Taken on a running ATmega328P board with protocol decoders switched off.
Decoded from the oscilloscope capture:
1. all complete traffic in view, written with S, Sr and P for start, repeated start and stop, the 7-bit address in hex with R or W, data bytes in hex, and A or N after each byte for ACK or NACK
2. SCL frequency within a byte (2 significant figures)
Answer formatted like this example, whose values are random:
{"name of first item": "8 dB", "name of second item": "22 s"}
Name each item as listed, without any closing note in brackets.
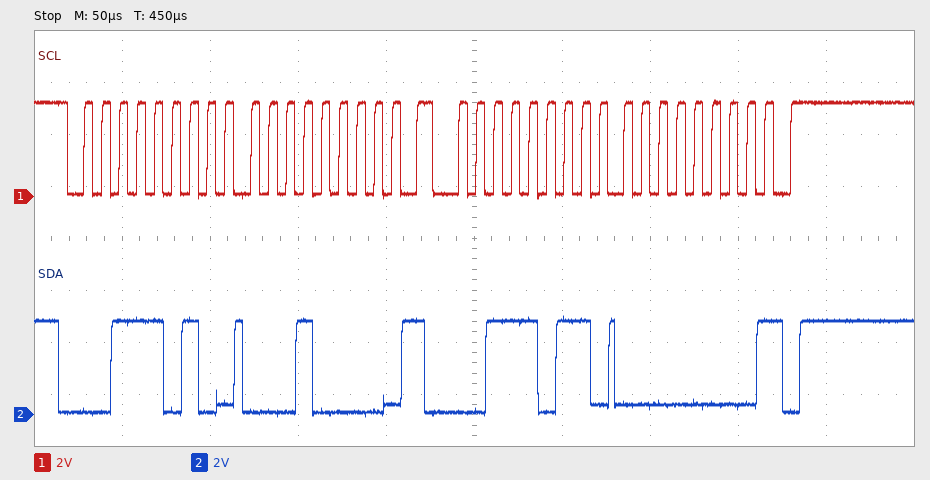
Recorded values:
{"all complete traffic in view, written with S, Sr and P for start, repeated start and stop, the 7-bit address in hex with R or W, data bytes in hex, and A or N after each byte for ACK or NACK": "S 1DW A 10 A Sr 1DR A 00 N P", "SCL frequency within a byte": "100 kHz"}
